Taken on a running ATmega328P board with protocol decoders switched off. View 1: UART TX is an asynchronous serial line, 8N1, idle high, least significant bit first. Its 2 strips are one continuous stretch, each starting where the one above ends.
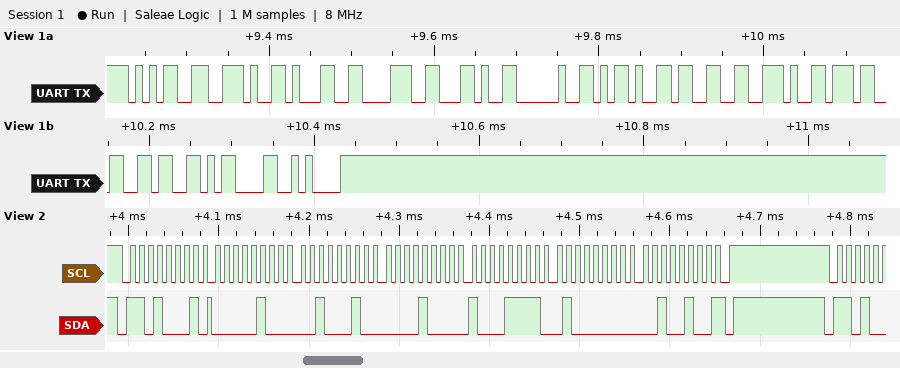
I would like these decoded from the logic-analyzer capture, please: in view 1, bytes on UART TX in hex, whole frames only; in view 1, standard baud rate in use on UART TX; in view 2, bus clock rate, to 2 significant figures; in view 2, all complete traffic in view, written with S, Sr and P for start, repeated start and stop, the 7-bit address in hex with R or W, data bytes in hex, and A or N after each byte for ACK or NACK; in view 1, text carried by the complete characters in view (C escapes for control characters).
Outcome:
35 2E 31 38 2C 20 2D 33 2E 37 36 0D 0A
115200 baud
100 kHz
S 68R A 04 A 22 A 08 A 8F A 40 A 24 N P
"5.18, -3.76\r\n"
